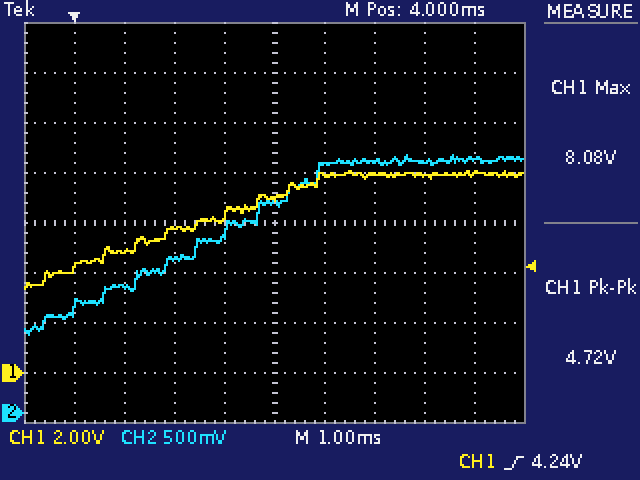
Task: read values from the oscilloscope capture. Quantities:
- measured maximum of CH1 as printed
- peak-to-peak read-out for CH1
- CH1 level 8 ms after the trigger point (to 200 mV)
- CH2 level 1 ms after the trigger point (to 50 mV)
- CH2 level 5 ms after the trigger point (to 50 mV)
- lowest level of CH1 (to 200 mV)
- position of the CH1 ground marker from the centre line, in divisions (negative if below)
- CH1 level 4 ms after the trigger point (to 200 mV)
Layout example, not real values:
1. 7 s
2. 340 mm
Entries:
1. 8.08 V
2. 4.72 V
3. 8.0 V
4. 1.25 V
5. 2.50 V
6. 3.4 V
7. -3.0 div
8. 7.0 V
